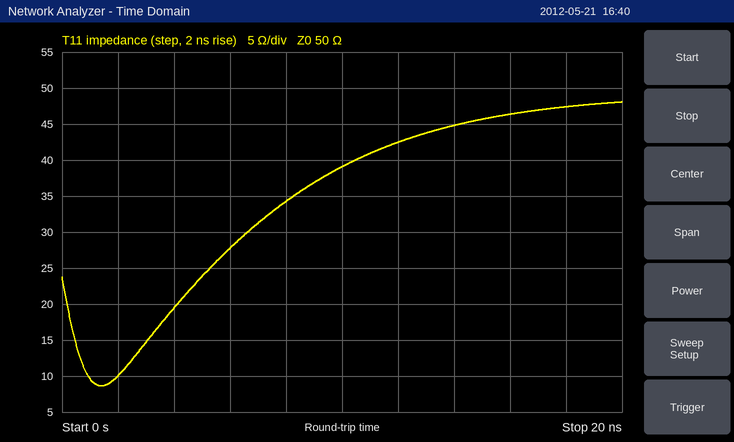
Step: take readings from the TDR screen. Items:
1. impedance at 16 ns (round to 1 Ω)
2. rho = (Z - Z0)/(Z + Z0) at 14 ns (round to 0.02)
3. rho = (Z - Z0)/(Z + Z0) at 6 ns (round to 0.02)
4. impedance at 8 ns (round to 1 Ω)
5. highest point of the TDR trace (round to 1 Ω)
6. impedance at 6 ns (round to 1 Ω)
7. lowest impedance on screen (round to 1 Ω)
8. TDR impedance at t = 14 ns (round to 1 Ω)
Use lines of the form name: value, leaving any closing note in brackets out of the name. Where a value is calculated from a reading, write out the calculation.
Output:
impedance at 16 ns: 46 Ω
rho = (Z - Z0)/(Z + Z0) at 14 ns: (45 − 50)/(45 + 50) ≈ -0.0526, so -0.06 to the nearest 0.02
rho = (Z - Z0)/(Z + Z0) at 6 ns: (28 − 50)/(28 + 50) ≈ -0.28
impedance at 8 ns: 34 Ω
highest point of the TDR trace: 48 Ω
impedance at 6 ns: 28 Ω
lowest impedance on screen: 9 Ω
TDR impedance at t = 14 ns: 45 Ω
